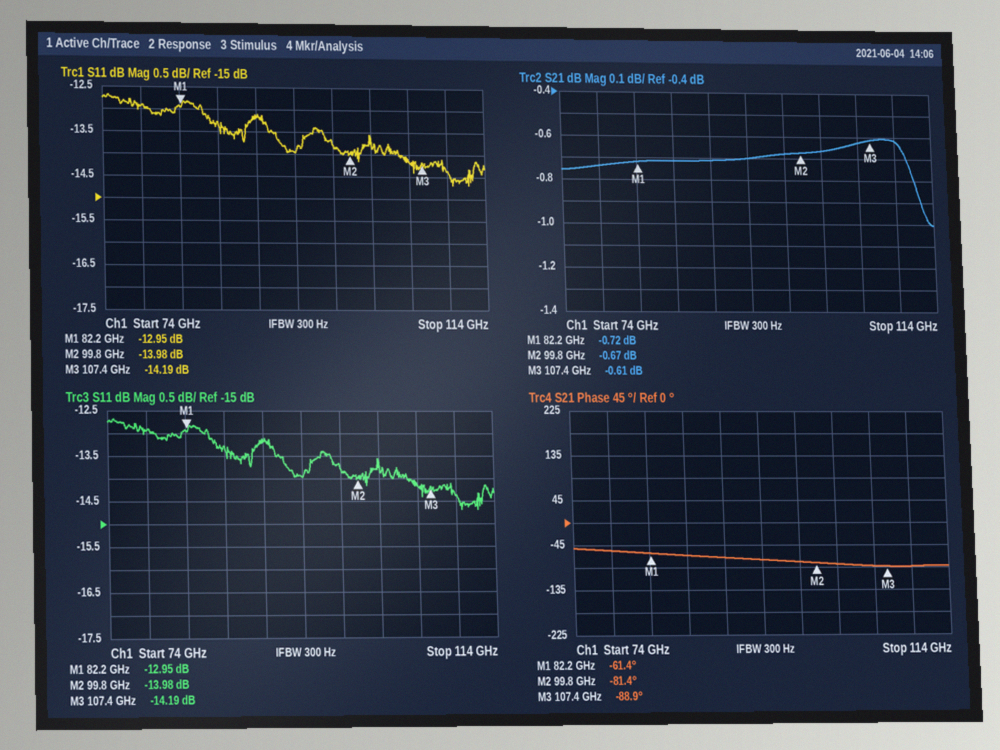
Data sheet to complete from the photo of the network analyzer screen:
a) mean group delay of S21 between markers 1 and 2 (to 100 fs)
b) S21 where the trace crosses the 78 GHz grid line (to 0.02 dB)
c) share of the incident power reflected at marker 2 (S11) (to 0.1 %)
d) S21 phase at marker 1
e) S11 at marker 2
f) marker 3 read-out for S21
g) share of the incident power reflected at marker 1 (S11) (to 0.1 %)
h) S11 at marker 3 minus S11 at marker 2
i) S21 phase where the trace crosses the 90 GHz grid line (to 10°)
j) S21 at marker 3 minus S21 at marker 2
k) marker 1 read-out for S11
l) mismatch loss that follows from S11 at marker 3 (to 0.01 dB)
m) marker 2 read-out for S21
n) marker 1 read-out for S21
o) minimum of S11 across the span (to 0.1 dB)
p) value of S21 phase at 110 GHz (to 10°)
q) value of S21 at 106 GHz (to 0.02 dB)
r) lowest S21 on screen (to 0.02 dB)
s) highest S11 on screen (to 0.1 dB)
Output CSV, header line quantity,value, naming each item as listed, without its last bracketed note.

quantity,value
mean group delay of S21 between markers 1 and 2,3.2 ps
S21 where the trace crosses the 78 GHz grid line,-0.74 dB
share of the incident power reflected at marker 2 (S11),4.0 %
S21 phase at marker 1,-61.4°
S11 at marker 2,-13.98 dB
marker 3 read-out for S21,-0.61 dB
share of the incident power reflected at marker 1 (S11),5.1 %
S11 at marker 3 minus S11 at marker 2,-0.21 dB
S21 phase where the trace crosses the 90 GHz grid line,-70°
S21 at marker 3 minus S21 at marker 2,0.06 dB
marker 1 read-out for S11,-12.95 dB
mismatch loss that follows from S11 at marker 3,0.17 dB
marker 2 read-out for S21,-0.67 dB
marker 1 read-out for S21,-0.72 dB
minimum of S11 across the span,-14.7 dB
value of S21 phase at 110 GHz,-90°
value of S21 at 106 GHz,-0.62 dB
lowest S21 on screen,-1.00 dB
highest S11 on screen,-12.7 dB
